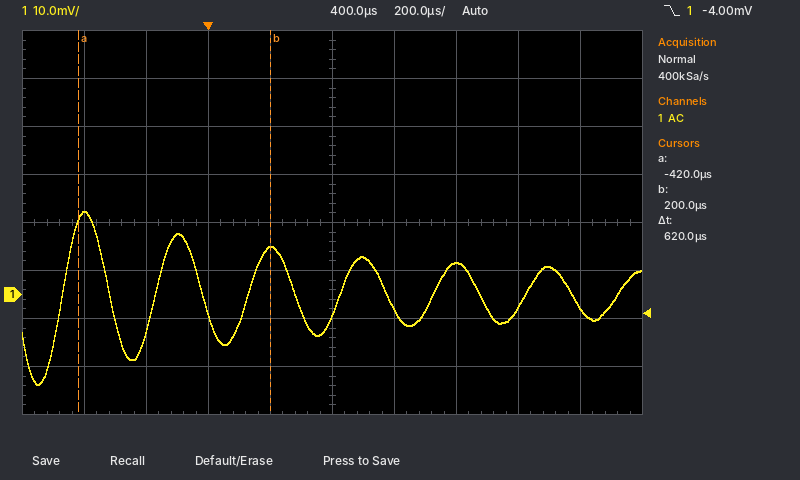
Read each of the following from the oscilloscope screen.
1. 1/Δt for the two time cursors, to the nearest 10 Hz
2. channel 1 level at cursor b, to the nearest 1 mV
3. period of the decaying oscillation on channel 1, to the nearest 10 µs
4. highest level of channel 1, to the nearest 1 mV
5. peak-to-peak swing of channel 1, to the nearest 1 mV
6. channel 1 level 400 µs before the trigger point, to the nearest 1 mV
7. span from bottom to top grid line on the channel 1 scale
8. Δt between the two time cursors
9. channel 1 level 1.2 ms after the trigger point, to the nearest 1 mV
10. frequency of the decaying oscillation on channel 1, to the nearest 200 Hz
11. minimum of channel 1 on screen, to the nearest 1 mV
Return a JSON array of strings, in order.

["1.61 kHz", "10 mV", "300 µs", "17 mV", "36 mV", "17 mV", "80 mV", "620 µs", "-3 mV", "3.4 kHz", "-19 mV"]
